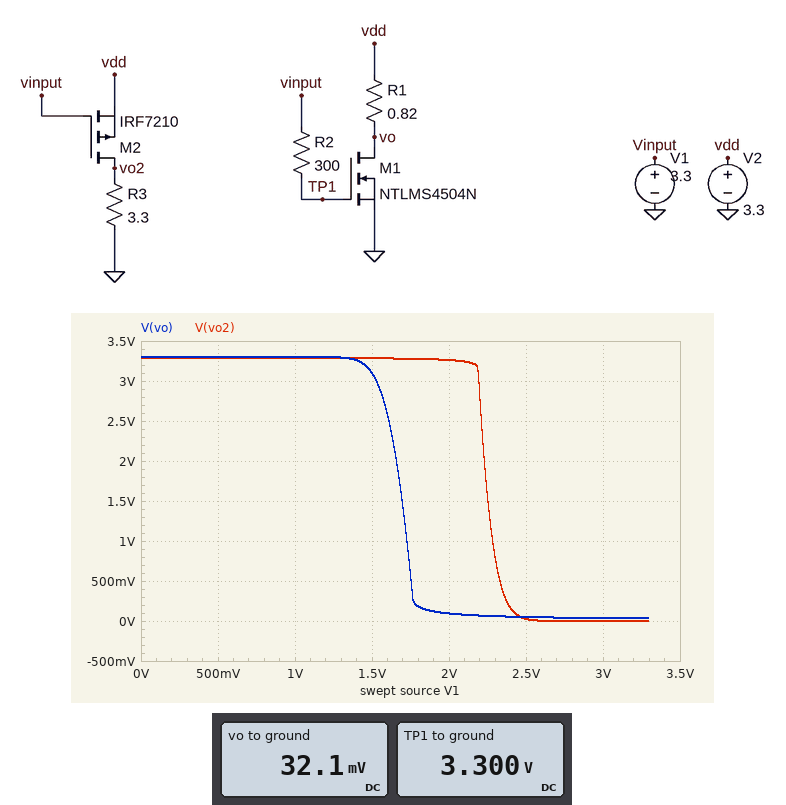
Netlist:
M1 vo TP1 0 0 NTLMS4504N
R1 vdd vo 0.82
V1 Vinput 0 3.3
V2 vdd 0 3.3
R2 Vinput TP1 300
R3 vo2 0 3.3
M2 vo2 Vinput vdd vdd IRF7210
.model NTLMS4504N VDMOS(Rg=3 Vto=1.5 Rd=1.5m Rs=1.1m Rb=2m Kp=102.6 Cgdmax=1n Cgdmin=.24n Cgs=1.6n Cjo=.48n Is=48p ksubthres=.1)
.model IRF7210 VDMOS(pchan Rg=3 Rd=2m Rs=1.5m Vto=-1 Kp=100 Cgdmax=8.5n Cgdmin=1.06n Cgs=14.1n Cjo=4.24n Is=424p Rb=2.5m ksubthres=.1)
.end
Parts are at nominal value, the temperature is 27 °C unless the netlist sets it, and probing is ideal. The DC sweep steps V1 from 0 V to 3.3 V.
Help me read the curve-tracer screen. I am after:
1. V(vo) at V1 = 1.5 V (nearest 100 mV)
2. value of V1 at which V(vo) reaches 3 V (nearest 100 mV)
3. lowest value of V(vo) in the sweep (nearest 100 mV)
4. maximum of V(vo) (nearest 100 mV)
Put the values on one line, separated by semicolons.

3.1 V; 1.5 V; 0 V; 3.3 V
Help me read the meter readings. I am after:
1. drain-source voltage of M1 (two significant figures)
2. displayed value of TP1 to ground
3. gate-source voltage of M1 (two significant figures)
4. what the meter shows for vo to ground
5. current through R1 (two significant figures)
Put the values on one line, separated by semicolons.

32 mV; 3.300 V; 3.3 V; 32.1 mV; 4.0 A
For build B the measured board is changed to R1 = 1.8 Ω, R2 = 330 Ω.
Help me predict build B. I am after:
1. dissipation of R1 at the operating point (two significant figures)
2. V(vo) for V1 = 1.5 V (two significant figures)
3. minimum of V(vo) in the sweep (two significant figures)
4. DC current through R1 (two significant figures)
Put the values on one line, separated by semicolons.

6.0 W; 2.9 V; 15 mV; 1.8 A
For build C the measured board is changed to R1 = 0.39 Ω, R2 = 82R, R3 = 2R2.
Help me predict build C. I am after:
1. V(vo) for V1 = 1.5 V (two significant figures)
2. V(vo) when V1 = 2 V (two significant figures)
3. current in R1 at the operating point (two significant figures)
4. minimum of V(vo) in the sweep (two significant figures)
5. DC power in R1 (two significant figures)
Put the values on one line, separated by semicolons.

3.2 V; 220 mV; 8.3 A; 67 mV; 27 W
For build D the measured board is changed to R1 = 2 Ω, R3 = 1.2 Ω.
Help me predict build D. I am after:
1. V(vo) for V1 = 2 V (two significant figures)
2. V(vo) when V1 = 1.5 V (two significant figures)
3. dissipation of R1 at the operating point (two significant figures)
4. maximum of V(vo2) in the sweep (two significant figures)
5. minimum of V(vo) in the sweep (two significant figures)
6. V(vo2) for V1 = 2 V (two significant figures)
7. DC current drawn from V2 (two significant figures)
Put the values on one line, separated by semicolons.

37 mV; 2.8 V; 5.4 W; 3.3 V; 13 mV; 3.2 V; 1.6 A
